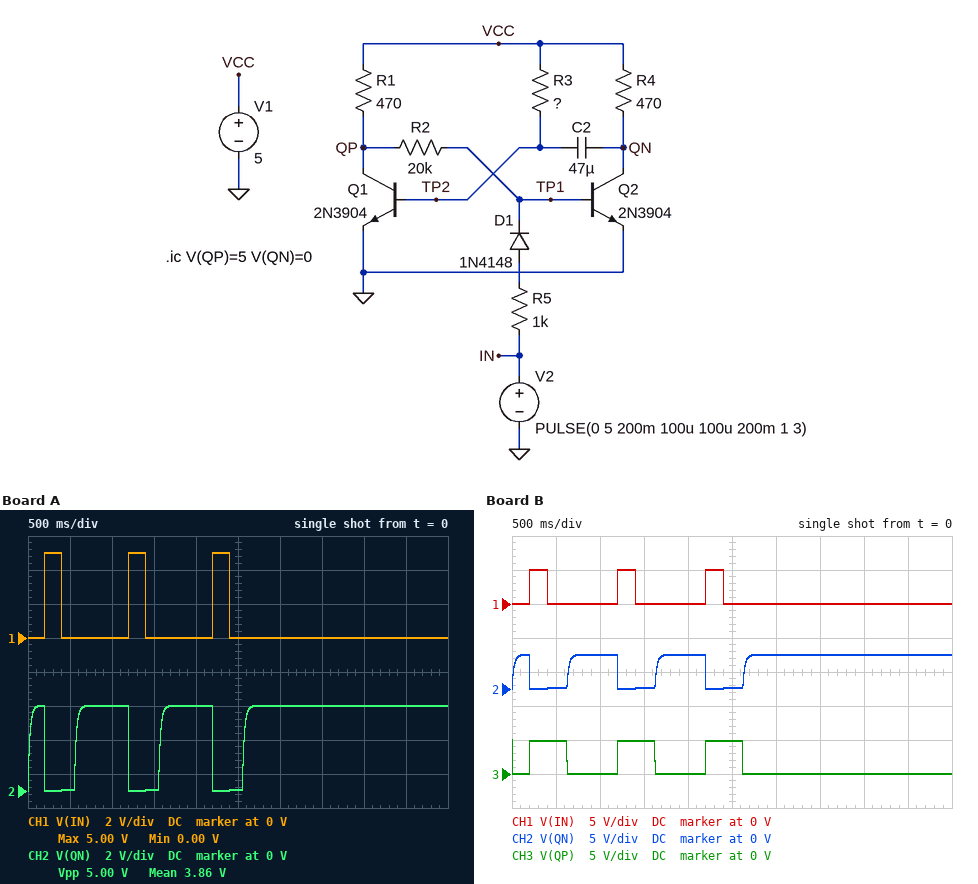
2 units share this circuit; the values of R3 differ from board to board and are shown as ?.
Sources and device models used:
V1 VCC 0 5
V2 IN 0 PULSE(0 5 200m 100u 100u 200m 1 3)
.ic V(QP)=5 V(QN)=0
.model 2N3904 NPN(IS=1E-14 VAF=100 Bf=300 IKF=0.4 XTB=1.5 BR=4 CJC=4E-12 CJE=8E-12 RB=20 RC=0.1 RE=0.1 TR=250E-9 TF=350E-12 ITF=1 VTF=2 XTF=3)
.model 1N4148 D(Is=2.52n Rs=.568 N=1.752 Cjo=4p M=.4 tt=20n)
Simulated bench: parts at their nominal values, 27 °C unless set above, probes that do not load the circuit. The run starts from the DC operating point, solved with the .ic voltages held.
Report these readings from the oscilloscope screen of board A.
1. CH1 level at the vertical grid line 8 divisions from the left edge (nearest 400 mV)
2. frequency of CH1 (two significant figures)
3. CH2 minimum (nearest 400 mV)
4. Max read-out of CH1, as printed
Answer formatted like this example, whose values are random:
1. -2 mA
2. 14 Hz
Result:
1. 0 V
2. 1.0 Hz
3. 0 V
4. 5.00 V
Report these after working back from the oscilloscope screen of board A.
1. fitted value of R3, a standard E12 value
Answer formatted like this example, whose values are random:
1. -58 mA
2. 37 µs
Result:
1. 10 kΩ
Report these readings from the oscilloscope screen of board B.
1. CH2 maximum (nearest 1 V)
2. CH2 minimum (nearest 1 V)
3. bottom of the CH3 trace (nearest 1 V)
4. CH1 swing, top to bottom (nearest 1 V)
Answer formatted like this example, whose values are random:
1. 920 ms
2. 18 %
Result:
1. 5 V
2. 0 V
3. 0 V
4. 5 V
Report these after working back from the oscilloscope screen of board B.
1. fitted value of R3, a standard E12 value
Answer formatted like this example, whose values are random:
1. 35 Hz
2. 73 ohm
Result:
1. 12 kΩ
